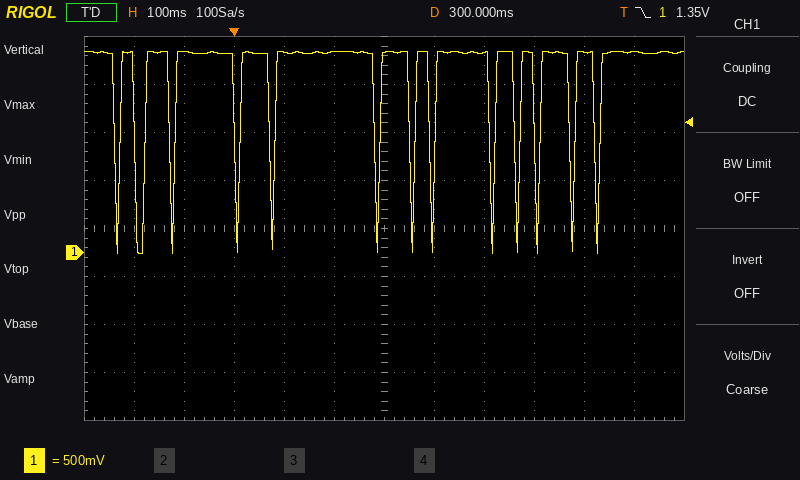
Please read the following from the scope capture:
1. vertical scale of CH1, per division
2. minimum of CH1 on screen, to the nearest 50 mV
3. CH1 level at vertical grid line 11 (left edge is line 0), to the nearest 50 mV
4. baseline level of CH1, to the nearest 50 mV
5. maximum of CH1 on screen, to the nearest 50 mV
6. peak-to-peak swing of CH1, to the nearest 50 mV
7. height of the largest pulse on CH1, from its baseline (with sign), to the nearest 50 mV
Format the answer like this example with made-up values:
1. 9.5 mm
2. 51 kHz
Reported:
1. 500 mV
2. 0 mV
3. 2.10 V
4. 2.10 V
5. 2.10 V
6. 2.10 V
7. -2.10 V
